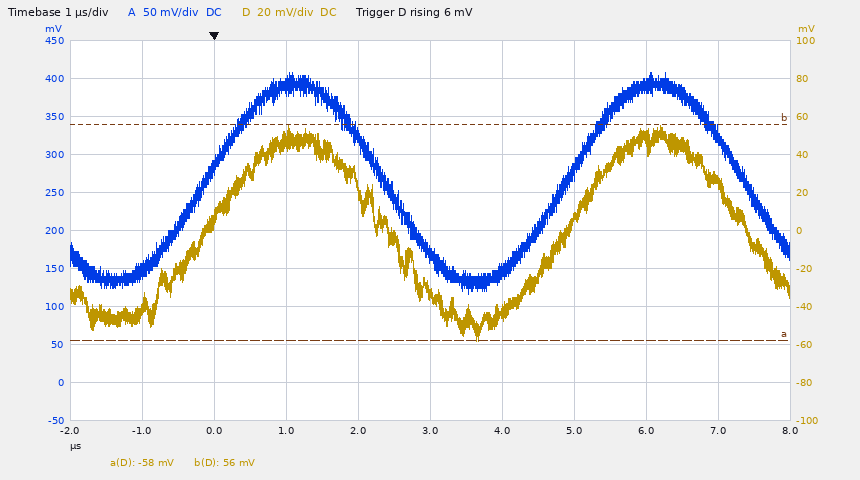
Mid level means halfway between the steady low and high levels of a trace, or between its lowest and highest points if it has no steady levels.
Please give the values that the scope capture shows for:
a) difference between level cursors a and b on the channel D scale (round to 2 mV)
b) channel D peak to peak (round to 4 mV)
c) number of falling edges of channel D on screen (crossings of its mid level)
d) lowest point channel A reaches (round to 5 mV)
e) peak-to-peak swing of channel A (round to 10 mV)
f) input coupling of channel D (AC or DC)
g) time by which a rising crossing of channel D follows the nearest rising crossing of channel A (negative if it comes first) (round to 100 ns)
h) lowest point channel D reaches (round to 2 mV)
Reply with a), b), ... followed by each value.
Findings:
a) 114 mV
b) 112 mV
c) 2
d) 115 mV
e) 290 mV
f) DC
g) 0.0 µs
h) -58 mV
